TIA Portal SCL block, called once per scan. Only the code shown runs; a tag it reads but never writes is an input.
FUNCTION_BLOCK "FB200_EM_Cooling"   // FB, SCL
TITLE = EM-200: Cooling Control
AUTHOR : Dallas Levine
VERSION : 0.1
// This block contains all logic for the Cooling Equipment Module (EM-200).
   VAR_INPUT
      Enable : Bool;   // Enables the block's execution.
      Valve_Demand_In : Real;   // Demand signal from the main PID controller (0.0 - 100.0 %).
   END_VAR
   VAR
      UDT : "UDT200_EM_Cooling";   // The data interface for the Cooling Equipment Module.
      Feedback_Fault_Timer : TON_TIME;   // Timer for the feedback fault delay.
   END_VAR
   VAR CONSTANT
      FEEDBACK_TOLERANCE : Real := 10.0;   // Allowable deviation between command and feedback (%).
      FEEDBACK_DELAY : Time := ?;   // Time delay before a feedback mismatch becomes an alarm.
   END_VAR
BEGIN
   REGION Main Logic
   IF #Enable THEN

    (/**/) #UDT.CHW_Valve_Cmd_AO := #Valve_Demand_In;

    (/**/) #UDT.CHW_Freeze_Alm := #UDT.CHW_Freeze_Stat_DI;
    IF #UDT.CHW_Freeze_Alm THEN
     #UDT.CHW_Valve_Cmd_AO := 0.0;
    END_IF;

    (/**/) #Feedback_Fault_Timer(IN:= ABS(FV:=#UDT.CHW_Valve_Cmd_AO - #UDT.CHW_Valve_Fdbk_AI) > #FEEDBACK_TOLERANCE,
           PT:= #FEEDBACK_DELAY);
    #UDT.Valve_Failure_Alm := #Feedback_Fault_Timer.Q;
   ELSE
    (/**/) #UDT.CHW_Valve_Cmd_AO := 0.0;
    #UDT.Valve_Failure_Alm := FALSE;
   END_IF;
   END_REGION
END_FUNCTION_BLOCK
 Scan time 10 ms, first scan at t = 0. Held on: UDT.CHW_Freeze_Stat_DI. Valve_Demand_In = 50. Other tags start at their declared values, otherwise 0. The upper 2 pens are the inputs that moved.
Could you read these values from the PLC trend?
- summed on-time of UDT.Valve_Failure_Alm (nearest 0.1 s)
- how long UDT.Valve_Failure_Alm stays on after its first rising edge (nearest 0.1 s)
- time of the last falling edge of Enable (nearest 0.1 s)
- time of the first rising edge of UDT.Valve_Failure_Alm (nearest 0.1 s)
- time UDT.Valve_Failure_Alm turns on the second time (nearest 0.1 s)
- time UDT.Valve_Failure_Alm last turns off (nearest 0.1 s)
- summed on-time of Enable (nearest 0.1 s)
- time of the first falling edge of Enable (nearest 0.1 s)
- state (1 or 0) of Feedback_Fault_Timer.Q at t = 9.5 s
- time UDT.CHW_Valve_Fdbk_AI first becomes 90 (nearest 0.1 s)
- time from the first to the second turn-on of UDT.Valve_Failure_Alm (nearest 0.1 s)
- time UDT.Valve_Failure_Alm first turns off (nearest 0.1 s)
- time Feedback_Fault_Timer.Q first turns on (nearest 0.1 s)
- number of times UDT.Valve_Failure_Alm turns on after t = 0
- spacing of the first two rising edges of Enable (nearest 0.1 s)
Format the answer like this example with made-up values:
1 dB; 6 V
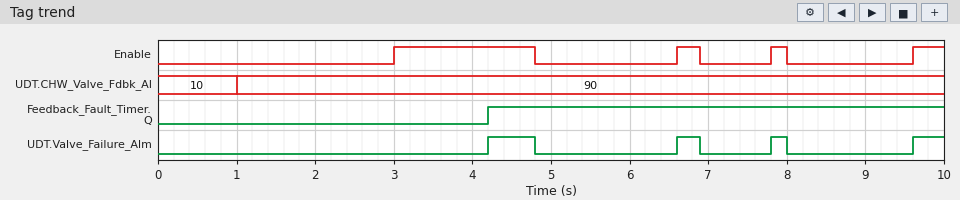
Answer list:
1.5 s; 0.6 s; 8.0 s; 4.2 s; 6.6 s; 8.0 s; 2.7 s; 4.8 s; 1; 1.0 s; 2.4 s; 4.8 s; 4.2 s; 4; 3.6 s
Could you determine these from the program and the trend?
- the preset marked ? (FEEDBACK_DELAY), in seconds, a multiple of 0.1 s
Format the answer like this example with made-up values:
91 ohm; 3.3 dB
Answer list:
1.2 s
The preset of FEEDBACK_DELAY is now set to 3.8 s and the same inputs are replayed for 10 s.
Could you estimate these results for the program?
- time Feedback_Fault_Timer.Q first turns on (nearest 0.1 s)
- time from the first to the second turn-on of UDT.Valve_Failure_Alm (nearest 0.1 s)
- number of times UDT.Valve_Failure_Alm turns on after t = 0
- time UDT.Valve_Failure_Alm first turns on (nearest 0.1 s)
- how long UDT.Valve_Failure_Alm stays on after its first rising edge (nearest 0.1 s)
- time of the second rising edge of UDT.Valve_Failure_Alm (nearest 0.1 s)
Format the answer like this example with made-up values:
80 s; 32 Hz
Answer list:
6.8 s; 1.0 s; 3; 6.8 s; 0.1 s; 7.8 s
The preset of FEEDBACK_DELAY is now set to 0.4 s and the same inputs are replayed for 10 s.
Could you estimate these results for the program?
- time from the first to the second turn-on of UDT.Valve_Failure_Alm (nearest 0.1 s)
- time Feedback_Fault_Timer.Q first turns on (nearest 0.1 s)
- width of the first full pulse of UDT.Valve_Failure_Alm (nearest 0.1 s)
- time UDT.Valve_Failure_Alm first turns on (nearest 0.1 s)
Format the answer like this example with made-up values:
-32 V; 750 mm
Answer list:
3.2 s; 3.4 s; 1.4 s; 3.4 s
